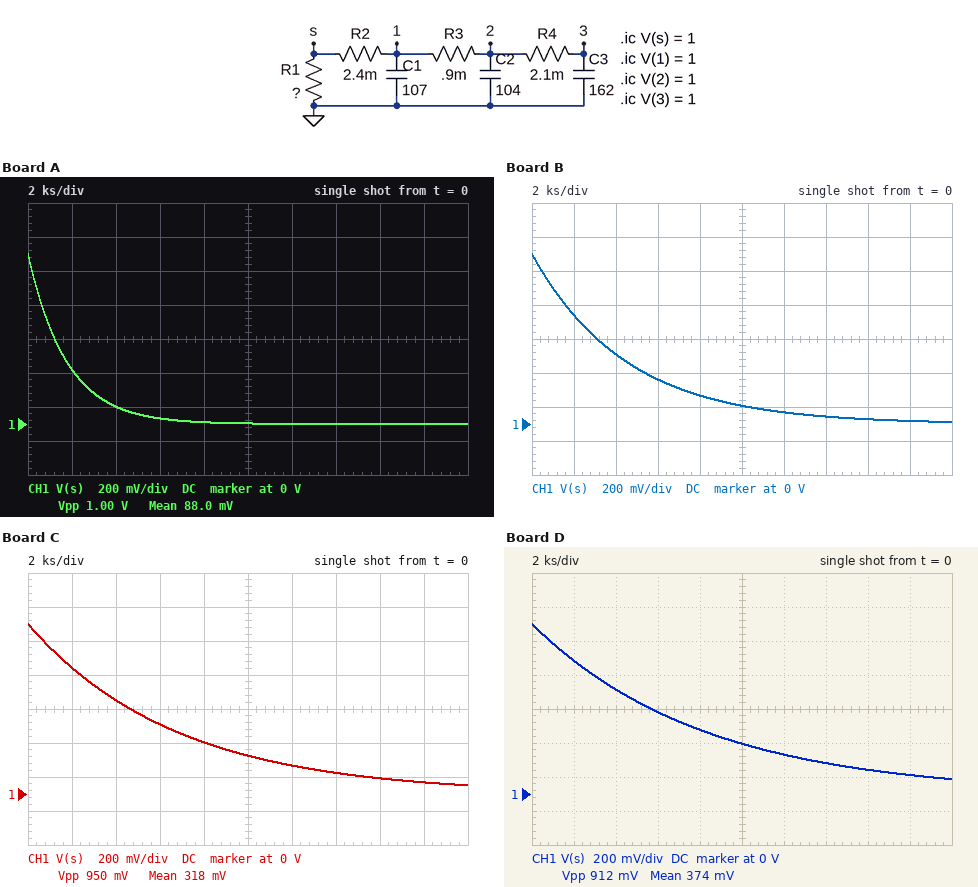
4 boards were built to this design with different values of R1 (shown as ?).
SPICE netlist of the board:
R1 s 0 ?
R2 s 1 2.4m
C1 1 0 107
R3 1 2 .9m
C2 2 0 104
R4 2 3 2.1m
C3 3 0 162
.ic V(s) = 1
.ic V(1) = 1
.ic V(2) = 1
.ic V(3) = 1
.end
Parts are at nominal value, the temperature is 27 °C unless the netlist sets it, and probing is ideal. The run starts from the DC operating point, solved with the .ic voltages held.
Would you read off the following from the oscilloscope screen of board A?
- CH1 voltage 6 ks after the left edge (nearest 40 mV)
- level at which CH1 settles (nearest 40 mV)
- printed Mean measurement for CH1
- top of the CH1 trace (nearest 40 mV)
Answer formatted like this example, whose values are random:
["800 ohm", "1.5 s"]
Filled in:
["40 mV", "0 V", "88.0 mV", "1.00 V"]
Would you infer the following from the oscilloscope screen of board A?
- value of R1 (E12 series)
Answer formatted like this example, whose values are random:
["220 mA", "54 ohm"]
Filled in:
["4.7 Ω"]
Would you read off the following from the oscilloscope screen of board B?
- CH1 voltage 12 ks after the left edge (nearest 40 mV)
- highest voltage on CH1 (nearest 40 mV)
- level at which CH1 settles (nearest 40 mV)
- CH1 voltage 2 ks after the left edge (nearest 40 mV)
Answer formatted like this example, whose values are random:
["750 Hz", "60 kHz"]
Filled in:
["80 mV", "1.00 V", "0 V", "640 mV"]
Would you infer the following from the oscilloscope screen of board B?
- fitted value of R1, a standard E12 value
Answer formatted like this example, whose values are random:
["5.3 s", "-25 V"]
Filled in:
["12 Ω"]
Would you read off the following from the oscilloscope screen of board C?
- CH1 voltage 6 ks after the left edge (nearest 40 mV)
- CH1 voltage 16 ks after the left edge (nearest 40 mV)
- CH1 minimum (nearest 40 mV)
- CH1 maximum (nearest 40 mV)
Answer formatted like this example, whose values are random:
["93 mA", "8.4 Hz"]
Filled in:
["400 mV", "80 mV", "40 mV", "1.00 V"]
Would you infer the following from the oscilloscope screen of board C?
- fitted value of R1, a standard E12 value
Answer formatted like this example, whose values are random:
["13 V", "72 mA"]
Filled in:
["18 Ω"]
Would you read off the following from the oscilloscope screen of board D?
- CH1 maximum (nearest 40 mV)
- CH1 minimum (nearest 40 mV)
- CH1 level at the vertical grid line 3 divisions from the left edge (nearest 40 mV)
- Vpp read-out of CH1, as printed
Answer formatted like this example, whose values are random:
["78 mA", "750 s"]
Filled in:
["1.00 V", "80 mV", "480 mV", "912 mV"]
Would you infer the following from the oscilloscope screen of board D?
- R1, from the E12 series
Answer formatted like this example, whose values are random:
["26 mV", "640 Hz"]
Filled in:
["22 Ω"]
